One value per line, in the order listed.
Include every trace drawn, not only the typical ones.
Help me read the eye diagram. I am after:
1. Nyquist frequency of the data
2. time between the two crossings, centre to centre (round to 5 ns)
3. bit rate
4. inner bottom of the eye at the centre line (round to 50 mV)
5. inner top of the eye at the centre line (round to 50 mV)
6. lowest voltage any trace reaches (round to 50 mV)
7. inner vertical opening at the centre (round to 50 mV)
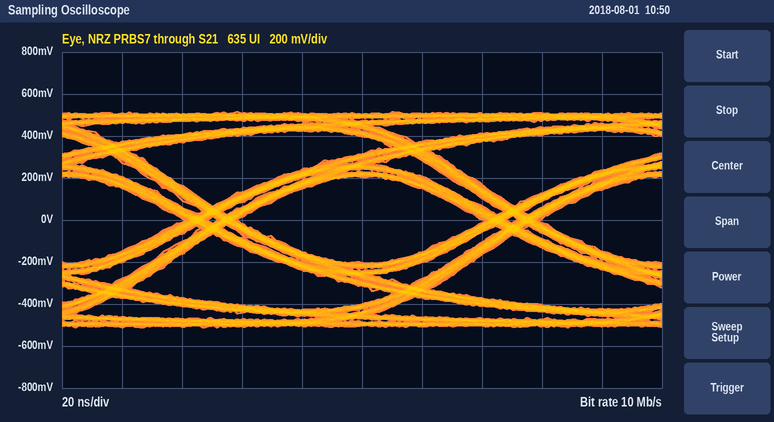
5 MHz
100 ns
10 Mb/s
-200 mV
200 mV
-500 mV
400 mV
